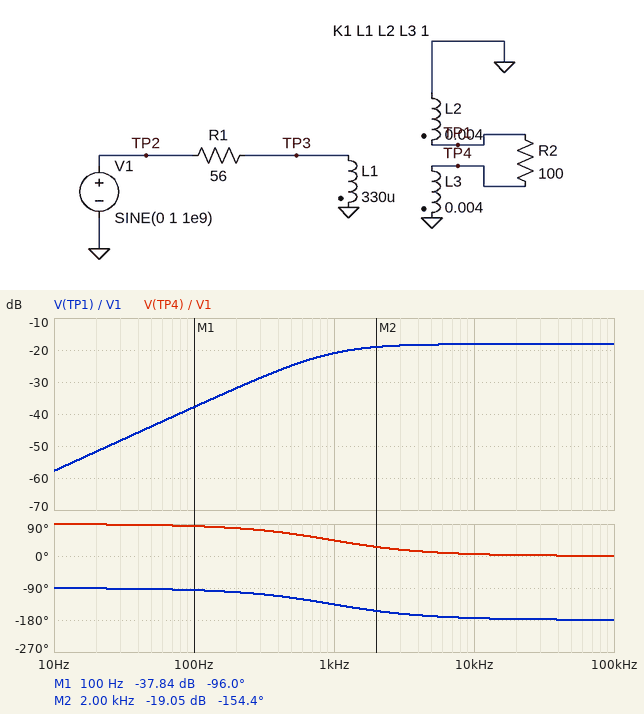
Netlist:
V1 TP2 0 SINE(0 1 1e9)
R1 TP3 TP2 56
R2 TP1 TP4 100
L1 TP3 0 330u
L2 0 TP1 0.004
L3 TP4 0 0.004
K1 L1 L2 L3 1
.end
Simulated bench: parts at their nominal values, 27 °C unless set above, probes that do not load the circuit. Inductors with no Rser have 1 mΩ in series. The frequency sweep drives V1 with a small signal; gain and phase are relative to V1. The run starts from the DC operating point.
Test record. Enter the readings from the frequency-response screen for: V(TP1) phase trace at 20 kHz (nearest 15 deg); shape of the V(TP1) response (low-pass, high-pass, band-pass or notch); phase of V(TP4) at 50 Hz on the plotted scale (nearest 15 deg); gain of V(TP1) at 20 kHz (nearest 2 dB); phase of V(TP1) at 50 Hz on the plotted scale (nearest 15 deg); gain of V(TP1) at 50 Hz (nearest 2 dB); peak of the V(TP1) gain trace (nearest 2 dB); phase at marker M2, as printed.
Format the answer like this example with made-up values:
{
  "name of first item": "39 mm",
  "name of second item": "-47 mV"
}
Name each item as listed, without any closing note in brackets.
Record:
{
  "V(TP1) phase trace at 20 kHz": "-180 deg",
  "shape of the V(TP1) response": "high-pass",
  "phase of V(TP4) at 50 Hz on the plotted scale": "90 deg",
  "gain of V(TP1) at 20 kHz": "-18 dB",
  "phase of V(TP1) at 50 Hz on the plotted scale": "-90 deg",
  "gain of V(TP1) at 50 Hz": "-44 dB",
  "peak of the V(TP1) gain trace": "-18 dB",
  "phase at marker M2, as printed": "-154.4 deg"
}
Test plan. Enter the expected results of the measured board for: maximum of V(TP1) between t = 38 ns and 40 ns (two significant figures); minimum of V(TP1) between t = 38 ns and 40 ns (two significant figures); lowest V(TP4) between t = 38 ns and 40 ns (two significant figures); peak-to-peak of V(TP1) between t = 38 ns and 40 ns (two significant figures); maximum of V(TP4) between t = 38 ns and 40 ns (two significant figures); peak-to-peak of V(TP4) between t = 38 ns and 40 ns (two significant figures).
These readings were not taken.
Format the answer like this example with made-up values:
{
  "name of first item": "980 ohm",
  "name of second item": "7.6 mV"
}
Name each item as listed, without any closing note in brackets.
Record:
{
  "maximum of V(TP1) between t = 38 ns and 40 ns": "120 mV",
  "minimum of V(TP1) between t = 38 ns and 40 ns": "-120 mV",
  "lowest V(TP4) between t = 38 ns and 40 ns": "-120 mV",
  "peak-to-peak of V(TP1) between t = 38 ns and 40 ns": "250 mV",
  "maximum of V(TP4) between t = 38 ns and 40 ns": "120 mV",
  "peak-to-peak of V(TP4) between t = 38 ns and 40 ns": "250 mV"
}
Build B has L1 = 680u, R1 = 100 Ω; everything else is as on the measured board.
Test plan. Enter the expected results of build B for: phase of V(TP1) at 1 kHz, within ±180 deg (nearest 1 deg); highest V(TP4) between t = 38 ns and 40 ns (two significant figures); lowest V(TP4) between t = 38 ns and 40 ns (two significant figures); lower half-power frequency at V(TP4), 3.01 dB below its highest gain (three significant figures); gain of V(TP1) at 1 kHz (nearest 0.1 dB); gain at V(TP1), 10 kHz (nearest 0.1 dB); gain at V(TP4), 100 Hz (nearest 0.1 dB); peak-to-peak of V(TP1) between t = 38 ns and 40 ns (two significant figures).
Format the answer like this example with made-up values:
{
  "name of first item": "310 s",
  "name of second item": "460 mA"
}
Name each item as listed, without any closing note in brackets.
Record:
{
  "phase of V(TP1) at 1 kHz, within ±180 deg": "-136 deg",
  "highest V(TP4) between t = 38 ns and 40 ns": "99 mV",
  "lowest V(TP4) between t = 38 ns and 40 ns": "-99 mV",
  "lower half-power frequency at V(TP4), 3.01 dB below its highest gain": "954 Hz",
  "gain of V(TP1) at 1 kHz": "-22.9 dB",
  "gain at V(TP1), 10 kHz": "-20.1 dB",
  "gain at V(TP4), 100 Hz": "-39.7 dB",
  "peak-to-peak of V(TP1) between t = 38 ns and 40 ns": "200 mV"
}
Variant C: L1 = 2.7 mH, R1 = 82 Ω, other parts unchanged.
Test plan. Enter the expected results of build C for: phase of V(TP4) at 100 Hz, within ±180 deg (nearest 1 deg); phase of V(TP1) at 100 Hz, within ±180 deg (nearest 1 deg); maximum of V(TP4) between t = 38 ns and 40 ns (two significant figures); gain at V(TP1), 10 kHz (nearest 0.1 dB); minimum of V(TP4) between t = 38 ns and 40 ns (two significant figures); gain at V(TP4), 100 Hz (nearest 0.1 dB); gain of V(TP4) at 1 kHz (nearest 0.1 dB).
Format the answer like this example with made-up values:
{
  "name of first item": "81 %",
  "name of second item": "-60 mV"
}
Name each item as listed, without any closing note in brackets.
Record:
{
  "phase of V(TP4) at 100 Hz, within ±180 deg": "83 deg",
  "phase of V(TP1) at 100 Hz, within ±180 deg": "-97 deg",
  "maximum of V(TP4) between t = 38 ns and 40 ns": "210 mV",
  "gain at V(TP1), 10 kHz": "-13.7 dB",
  "minimum of V(TP4) between t = 38 ns and 40 ns": "-210 mV",
  "gain at V(TP4), 100 Hz": "-32.0 dB",
  "gain of V(TP4) at 1 kHz": "-15.9 dB"
}
